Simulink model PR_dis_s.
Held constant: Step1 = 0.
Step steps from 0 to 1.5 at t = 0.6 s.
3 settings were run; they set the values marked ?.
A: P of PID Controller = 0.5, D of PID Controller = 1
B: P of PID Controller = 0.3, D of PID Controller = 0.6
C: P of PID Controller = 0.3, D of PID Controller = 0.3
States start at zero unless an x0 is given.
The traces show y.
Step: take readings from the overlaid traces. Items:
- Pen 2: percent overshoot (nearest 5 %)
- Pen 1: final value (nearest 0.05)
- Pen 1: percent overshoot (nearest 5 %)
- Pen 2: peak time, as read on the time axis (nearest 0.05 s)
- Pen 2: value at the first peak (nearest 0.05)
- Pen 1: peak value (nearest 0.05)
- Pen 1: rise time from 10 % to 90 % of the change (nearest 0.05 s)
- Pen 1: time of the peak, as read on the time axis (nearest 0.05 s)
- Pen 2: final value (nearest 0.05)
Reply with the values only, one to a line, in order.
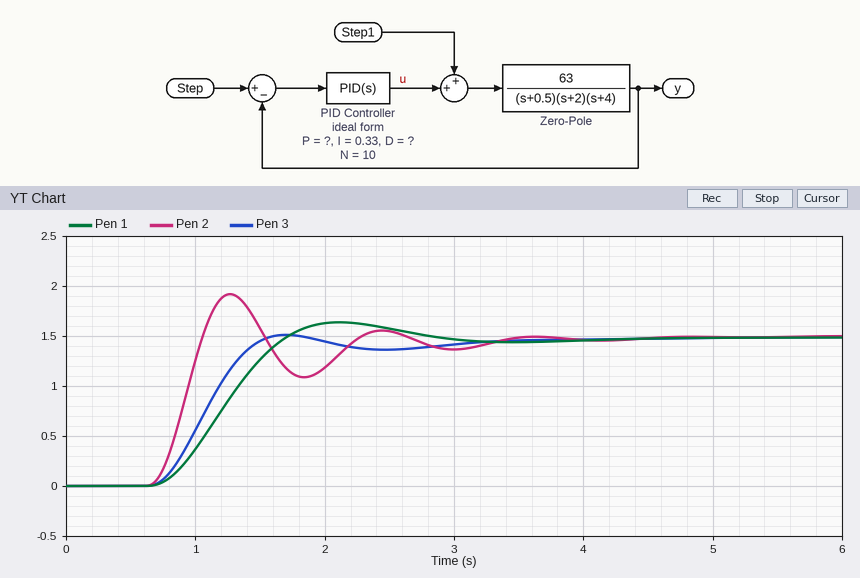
30 %
1.50
10 %
1.25 s
1.90
1.65
0.70 s
2.10 s
1.50
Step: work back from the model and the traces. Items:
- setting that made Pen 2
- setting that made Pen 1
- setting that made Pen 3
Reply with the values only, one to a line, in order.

A
C
B
